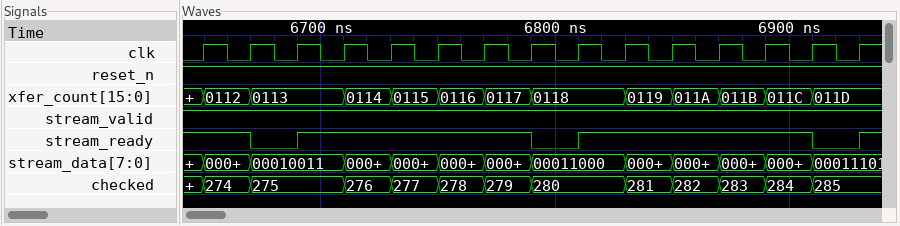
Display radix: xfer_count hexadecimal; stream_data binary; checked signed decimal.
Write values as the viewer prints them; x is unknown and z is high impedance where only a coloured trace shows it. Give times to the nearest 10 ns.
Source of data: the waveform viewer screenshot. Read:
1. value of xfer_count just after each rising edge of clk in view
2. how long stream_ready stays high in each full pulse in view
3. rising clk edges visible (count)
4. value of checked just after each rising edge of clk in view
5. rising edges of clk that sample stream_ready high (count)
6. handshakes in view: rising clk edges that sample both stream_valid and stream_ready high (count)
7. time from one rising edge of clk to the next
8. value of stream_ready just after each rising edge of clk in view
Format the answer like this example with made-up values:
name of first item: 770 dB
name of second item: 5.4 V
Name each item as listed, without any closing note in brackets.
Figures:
value of xfer_count just after each rising edge of clk in view: 0112, 0113, 0113, 0114, 0115, 0116, 0117, 0118, 0118, 0119, 011A, 011B, 011C, 011D, 011D
how long stream_ready stays high in each full pulse in view: 100 ns, 100 ns
rising clk edges visible: 15
value of checked just after each rising edge of clk in view: 274, 275, 275, 276, 277, 278, 279, 280, 280, 281, 282, 283, 284, 285, 285
rising edges of clk that sample stream_ready high: 12
handshakes in view: rising clk edges that sample both stream_valid and stream_ready high: 12
time from one rising edge of clk to the next: 20 ns
value of stream_ready just after each rising edge of clk in view: 1 0 1 1 1 1 1 0 1 1 1 1 1 0 1
